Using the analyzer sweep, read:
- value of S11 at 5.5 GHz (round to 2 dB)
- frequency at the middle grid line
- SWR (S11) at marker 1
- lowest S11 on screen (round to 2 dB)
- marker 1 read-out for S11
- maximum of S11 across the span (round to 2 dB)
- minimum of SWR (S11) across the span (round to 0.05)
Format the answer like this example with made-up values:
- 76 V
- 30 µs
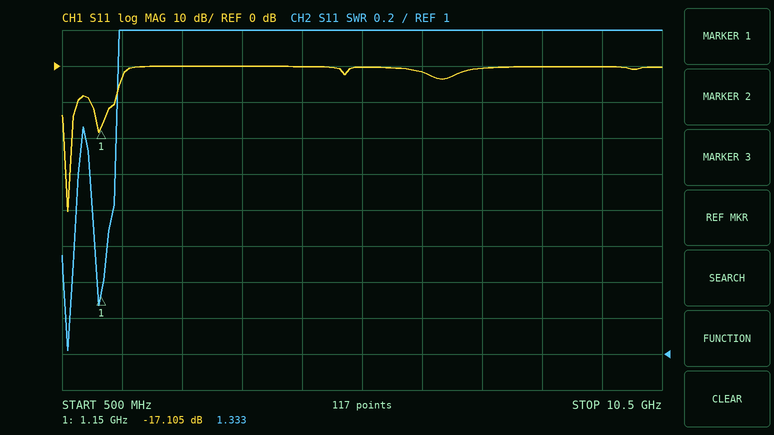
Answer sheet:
- 0 dB
- 5.5 GHz
- 1.333
- -40 dB
- -17.105 dB
- 0 dB
- 1.00
